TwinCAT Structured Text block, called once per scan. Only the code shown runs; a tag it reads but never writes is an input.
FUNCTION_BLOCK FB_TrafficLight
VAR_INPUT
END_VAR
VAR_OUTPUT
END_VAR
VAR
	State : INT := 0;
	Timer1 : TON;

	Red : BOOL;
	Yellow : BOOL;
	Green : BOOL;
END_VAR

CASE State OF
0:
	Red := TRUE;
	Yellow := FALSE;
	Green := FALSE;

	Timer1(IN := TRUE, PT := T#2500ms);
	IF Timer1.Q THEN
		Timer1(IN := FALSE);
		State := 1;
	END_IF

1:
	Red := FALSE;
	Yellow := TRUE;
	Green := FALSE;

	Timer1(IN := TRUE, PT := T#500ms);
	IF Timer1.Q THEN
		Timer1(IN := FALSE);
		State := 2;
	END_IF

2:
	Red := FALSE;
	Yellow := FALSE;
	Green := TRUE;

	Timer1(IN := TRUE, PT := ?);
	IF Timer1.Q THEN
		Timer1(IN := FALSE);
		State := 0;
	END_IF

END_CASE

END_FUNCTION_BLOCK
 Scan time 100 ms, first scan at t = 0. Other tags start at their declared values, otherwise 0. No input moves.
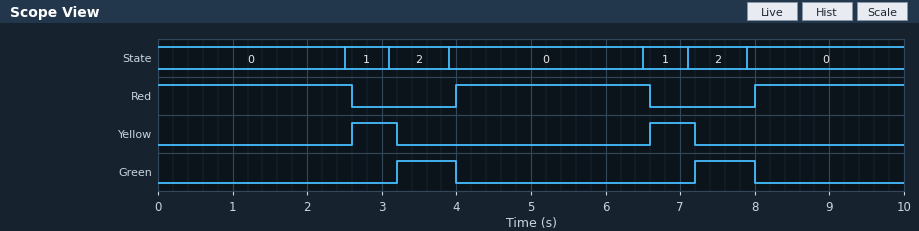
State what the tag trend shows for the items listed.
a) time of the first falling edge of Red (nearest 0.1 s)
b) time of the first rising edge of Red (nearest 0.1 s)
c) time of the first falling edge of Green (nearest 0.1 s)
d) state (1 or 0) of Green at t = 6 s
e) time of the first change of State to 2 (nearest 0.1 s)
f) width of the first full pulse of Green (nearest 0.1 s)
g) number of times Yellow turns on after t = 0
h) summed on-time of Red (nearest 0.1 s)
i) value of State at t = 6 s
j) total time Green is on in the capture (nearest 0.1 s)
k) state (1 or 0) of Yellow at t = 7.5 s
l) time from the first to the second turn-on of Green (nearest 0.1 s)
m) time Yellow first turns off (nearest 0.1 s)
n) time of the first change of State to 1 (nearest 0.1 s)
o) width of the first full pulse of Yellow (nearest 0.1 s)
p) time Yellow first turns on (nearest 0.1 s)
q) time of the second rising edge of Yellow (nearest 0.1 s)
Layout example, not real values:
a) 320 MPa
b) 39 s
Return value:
a) 2.6 s
b) 4.0 s
c) 4.0 s
d) 0
e) 3.1 s
f) 0.8 s
g) 2
h) 7.2 s
i) 0
j) 1.6 s
k) 0
l) 4.0 s
m) 3.2 s
n) 2.5 s
o) 0.6 s
p) 2.6 s
q) 6.6 s
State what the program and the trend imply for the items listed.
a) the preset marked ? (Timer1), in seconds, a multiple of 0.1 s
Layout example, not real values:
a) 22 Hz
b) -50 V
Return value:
a) 0.7 s
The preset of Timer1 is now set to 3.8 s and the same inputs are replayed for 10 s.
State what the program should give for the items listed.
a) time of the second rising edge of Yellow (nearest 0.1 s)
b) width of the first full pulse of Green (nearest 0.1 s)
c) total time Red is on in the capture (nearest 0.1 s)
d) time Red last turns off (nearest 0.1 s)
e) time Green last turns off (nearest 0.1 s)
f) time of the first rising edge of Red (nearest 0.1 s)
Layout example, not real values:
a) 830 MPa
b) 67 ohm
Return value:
a) 9.7 s
b) 3.9 s
c) 5.2 s
d) 9.7 s
e) 7.1 s
f) 7.1 s
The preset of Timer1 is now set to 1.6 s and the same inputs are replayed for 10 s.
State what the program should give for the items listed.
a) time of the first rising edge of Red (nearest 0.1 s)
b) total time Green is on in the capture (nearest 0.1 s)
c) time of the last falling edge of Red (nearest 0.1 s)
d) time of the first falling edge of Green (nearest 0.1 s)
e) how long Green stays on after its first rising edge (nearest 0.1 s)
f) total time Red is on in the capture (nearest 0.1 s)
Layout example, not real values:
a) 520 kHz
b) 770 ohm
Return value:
a) 4.9 s
b) 3.4 s
c) 7.5 s
d) 4.9 s
e) 1.7 s
f) 5.4 s
